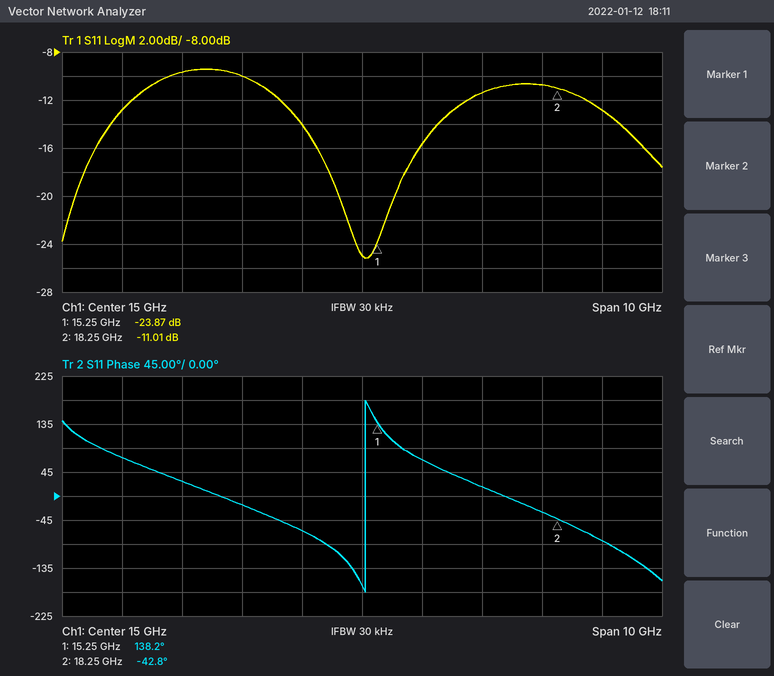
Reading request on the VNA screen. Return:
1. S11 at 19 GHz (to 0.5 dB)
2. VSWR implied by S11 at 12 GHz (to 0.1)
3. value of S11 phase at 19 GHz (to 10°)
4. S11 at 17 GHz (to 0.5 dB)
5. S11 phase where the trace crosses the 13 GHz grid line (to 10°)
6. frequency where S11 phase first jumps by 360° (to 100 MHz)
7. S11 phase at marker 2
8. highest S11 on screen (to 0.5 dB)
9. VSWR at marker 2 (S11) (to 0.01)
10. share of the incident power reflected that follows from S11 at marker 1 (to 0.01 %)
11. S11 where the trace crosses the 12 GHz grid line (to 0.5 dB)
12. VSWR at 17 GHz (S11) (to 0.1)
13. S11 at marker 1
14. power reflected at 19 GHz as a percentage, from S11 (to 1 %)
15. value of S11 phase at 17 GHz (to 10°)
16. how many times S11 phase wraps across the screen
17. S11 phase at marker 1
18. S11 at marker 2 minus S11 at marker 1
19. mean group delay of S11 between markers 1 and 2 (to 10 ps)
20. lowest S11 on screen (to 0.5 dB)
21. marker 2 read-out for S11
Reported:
-13.0 dB
2.0
-80°
-11.5 dB
-20°
15.1 GHz
-42.8°
-9.5 dB
1.78
0.41 %
-9.5 dB
1.7
-23.87 dB
5 %
20°
1
138.2°
12.86 dB
170 ps
-25.0 dB
-11.01 dB
